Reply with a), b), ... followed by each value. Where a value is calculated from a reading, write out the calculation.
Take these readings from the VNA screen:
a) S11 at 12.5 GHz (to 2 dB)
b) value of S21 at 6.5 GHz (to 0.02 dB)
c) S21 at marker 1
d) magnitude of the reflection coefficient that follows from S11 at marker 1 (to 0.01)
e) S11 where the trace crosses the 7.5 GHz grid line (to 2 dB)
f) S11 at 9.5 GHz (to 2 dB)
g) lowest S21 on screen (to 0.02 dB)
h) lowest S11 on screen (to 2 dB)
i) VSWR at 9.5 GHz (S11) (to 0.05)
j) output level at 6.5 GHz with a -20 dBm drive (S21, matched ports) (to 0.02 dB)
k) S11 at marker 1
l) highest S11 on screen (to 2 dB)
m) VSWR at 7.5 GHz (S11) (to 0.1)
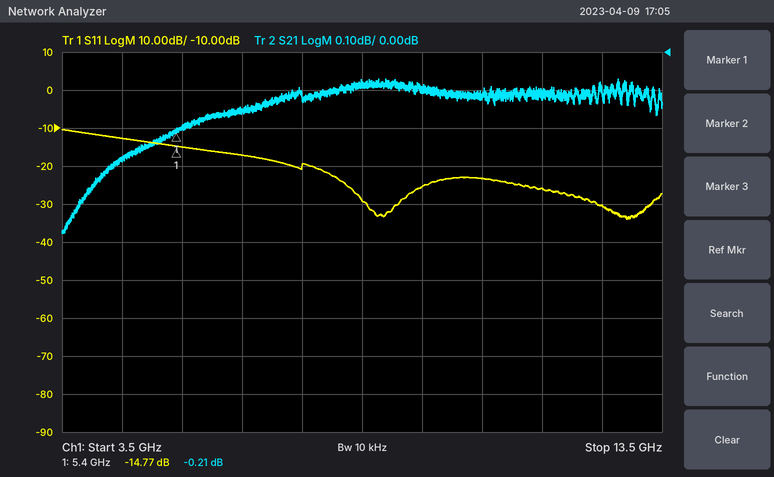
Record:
a) -30 dB
b) -0.16 dB
c) -0.21 dB
d) 10^(-14.77/20) ≈ 0.18
e) -20 dB
f) -26 dB
g) -0.48 dB
h) -34 dB
i) |Γ| = 10^(-26/20) = 0.0501; VSWR = (1 + 0.0501)/(1 − 0.0501) ≈ 1.11, so 1.10 to the nearest 0.05
j) -20 dBm + (-0.16 dB) = -20.16 dBm
k) -14.77 dB
l) -10 dB
m) |Γ| = 10^(-20/20) = 0.1000; VSWR = (1 + 0.1000)/(1 − 0.1000) ≈ 1.2
